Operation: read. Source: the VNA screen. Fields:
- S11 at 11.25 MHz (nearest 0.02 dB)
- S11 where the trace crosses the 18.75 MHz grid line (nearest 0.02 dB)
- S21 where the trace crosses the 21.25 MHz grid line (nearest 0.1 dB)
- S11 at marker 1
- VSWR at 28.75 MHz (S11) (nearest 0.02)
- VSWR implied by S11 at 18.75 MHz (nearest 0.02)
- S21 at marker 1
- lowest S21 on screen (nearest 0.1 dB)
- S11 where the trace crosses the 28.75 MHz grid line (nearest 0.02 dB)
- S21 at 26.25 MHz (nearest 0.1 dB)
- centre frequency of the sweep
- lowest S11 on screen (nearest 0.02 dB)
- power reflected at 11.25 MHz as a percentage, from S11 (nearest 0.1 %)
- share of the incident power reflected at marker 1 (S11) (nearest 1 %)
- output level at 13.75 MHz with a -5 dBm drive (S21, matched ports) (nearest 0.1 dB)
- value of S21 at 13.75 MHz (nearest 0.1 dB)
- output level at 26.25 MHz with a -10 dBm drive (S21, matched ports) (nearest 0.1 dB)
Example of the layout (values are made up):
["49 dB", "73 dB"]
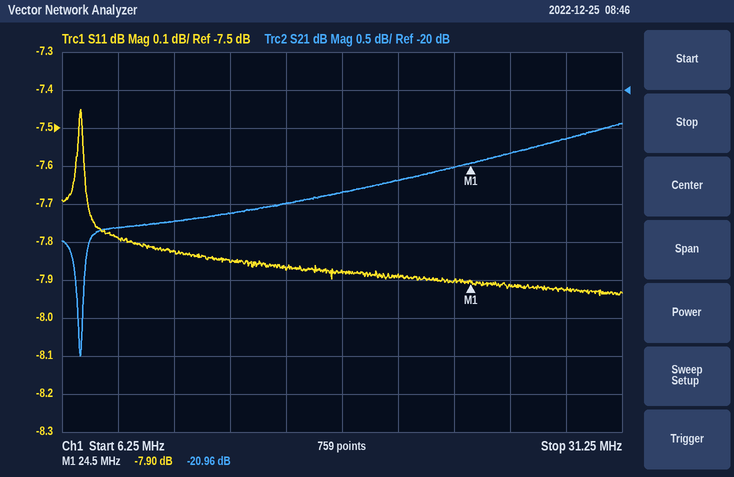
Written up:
["-7.82 dB", "-7.88 dB", "-21.2 dB", "-7.90 dB", "2.34", "2.36", "-20.96 dB", "-23.5 dB", "-7.92 dB", "-20.8 dB", "18.75 MHz", "-7.94 dB", "16.5 %", "16 %", "-26.6 dBm", "-21.6 dB", "-30.8 dBm"]
